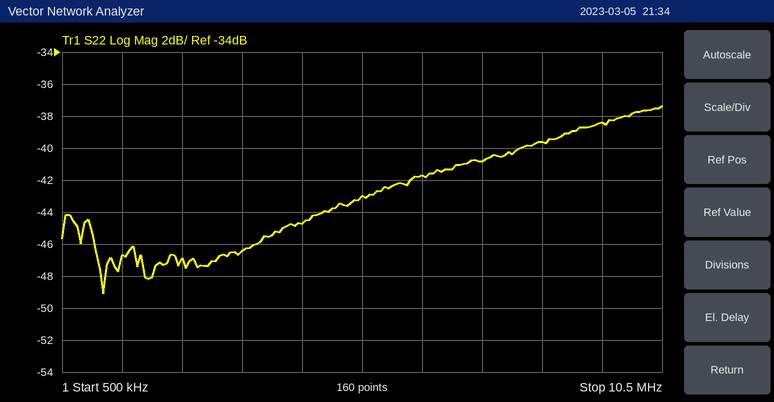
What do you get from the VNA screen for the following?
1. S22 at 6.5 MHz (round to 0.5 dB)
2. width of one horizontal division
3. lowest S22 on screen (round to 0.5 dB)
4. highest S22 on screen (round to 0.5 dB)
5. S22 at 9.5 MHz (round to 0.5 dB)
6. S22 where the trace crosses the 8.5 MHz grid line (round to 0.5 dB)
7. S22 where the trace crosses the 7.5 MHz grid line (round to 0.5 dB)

-41.5 dB
1 MHz
-49.0 dB
-37.5 dB
-38.5 dB
-39.5 dB
-41.0 dB
